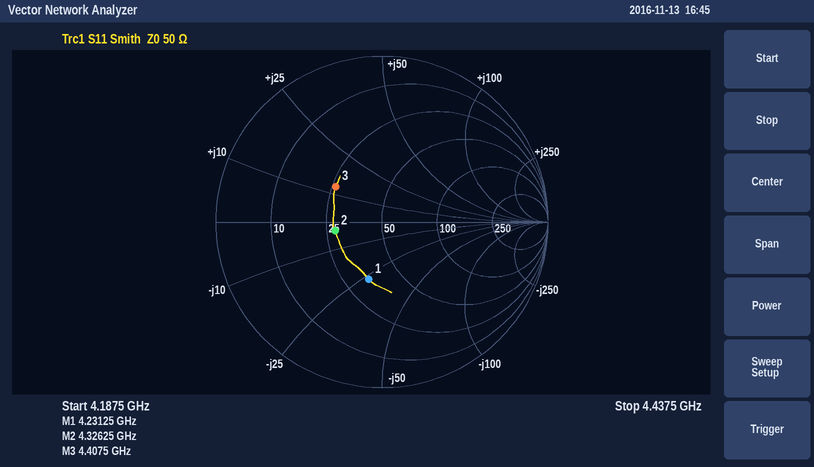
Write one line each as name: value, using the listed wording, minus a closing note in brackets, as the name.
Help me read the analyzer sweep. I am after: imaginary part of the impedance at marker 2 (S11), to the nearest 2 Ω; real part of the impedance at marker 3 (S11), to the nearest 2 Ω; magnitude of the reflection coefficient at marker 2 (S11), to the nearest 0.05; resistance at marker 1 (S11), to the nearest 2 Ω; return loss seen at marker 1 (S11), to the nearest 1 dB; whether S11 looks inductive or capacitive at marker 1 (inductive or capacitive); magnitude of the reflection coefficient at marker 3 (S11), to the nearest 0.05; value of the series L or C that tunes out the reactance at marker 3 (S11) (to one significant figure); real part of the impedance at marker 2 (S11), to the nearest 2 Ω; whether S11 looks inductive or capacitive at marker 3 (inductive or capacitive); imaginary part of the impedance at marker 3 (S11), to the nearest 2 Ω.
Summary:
imaginary part of the impedance at marker 2 (S11), to the nearest 2 Ω: -4 Ω
real part of the impedance at marker 3 (S11), to the nearest 2 Ω: 26 Ω
magnitude of the reflection coefficient at marker 2 (S11), to the nearest 0.05: 0.30
resistance at marker 1 (S11), to the nearest 2 Ω: 34 Ω
return loss seen at marker 1 (S11), to the nearest 1 dB: 9 dB
whether S11 looks inductive or capacitive at marker 1: capacitive
magnitude of the reflection coefficient at marker 3 (S11), to the nearest 0.05: 0.35
value of the series L or C that tunes out the reactance at marker 3 (S11): 3 pF
real part of the impedance at marker 2 (S11), to the nearest 2 Ω: 28 Ω
whether S11 looks inductive or capacitive at marker 3: inductive
imaginary part of the impedance at marker 3 (S11), to the nearest 2 Ω: +12 Ω
